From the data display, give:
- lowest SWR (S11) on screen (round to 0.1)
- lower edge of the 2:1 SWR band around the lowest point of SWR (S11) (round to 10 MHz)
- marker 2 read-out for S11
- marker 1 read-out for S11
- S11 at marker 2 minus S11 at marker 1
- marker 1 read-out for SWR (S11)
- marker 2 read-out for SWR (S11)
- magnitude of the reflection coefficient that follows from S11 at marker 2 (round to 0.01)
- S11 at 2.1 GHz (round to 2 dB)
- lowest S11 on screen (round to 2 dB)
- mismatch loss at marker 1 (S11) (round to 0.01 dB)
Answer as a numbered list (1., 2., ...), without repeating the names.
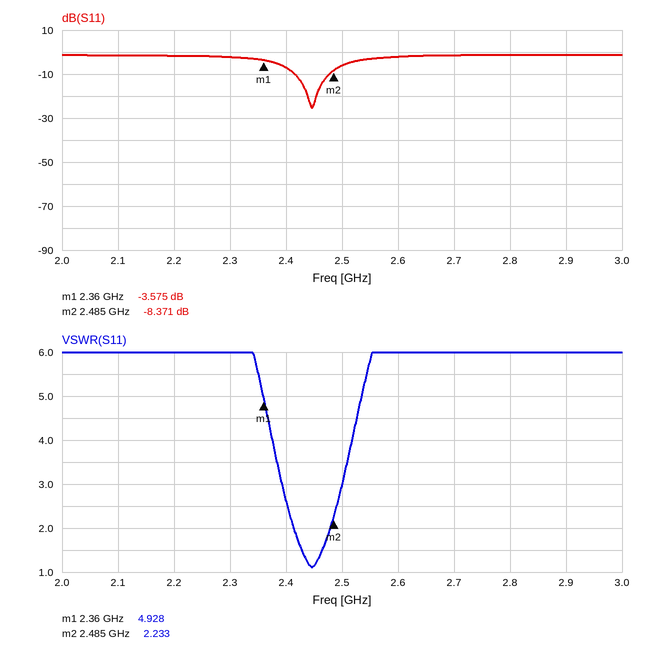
1. 1.1
2. 2.41 GHz
3. -8.371 dB
4. -3.575 dB
5. -4.796 dB
6. 4.928
7. 2.233
8. 0.38
9. -2 dB
10. -26 dB
11. 2.51 dB
